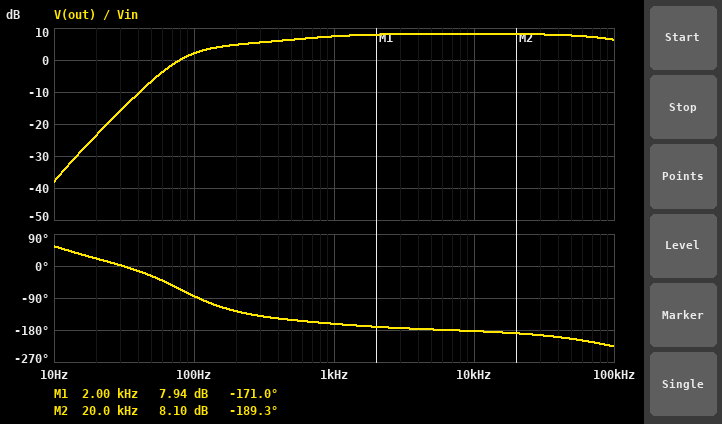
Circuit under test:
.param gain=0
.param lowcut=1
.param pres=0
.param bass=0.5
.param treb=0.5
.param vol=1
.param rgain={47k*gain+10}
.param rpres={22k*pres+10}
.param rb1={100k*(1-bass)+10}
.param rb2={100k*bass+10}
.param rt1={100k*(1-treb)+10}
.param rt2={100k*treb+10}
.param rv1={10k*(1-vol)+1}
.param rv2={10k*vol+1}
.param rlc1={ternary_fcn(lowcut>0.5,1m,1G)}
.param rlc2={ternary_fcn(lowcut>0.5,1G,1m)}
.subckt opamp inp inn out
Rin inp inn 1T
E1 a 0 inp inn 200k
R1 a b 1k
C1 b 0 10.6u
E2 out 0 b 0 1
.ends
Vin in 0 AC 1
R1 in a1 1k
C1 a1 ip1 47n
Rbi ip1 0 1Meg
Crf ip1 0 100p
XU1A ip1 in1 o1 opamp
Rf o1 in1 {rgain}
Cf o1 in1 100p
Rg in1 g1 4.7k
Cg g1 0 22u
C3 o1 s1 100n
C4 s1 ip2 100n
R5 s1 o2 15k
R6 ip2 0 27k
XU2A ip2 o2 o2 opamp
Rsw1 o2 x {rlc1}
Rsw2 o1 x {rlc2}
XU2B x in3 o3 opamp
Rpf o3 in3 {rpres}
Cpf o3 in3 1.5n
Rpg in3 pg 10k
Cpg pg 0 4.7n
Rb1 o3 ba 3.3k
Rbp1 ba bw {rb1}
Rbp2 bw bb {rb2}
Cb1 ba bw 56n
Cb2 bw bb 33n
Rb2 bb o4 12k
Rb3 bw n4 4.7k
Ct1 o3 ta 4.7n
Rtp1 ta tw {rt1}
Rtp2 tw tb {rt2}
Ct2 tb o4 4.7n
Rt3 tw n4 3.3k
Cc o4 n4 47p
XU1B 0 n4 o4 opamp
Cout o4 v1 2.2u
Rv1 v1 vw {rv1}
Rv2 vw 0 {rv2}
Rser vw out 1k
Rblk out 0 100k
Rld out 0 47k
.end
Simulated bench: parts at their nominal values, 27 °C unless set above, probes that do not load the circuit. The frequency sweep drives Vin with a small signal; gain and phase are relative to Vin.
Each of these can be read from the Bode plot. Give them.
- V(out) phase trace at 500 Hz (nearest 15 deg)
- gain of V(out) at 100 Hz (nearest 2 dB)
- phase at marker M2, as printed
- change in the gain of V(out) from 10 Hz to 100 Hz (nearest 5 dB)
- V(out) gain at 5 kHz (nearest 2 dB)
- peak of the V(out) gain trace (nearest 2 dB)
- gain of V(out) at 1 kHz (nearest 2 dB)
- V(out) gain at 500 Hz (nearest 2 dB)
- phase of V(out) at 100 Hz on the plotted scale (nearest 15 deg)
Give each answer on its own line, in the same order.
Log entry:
-150 deg
2 dB
-189.3 deg
40 dB
8 dB
8 dB
8 dB
6 dB
-90 deg
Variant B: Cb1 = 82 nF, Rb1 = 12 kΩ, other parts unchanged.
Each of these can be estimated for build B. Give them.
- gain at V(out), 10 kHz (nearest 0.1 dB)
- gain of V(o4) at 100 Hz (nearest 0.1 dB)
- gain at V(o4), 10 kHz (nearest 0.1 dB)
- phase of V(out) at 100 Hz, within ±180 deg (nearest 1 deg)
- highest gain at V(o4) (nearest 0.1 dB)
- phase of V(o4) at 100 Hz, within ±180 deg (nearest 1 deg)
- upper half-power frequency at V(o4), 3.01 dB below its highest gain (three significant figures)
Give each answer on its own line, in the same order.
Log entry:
-0.3 dB
2.7 dB
0 dB
-96 deg
4.0 dB
-101 deg
629 Hz
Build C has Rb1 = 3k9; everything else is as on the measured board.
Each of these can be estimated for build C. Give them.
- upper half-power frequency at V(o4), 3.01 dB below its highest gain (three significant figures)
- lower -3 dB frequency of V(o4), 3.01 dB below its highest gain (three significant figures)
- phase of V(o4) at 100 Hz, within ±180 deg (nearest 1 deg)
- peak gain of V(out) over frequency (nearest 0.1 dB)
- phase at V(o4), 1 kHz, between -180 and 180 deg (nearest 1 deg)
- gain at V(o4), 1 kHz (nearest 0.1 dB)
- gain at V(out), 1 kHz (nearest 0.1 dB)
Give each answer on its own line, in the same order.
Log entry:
146 kHz
158 Hz
-91 deg
7.1 dB
-166 deg
6.9 dB
6.6 dB
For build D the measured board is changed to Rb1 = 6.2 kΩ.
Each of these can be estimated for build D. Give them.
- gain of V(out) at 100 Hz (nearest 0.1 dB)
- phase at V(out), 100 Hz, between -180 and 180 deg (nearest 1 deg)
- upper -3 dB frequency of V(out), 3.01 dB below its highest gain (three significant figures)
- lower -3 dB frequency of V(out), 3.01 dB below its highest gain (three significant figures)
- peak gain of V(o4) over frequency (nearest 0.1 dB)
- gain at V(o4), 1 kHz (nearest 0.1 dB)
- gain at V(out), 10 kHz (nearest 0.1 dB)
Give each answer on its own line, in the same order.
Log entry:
1.5 dB
-89 deg
159 kHz
96.7 Hz
4.5 dB
4.4 dB
4.0 dB
